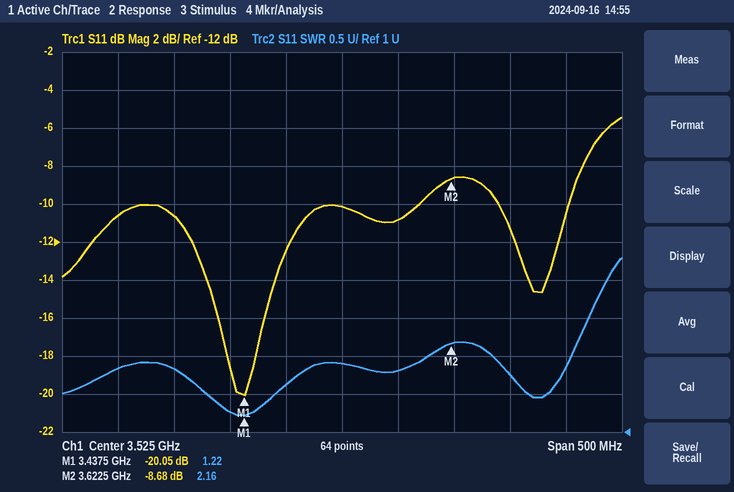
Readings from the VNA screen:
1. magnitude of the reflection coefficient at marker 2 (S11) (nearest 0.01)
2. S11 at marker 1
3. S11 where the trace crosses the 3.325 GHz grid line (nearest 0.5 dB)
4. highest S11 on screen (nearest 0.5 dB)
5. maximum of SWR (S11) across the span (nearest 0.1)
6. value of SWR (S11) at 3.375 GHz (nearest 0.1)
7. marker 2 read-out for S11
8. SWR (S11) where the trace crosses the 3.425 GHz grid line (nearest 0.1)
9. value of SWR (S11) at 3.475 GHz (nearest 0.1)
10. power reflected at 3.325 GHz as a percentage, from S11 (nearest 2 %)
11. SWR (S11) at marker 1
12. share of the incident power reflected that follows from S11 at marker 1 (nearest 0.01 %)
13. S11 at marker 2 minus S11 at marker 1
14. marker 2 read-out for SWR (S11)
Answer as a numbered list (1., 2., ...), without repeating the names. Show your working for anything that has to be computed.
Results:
1. 10^(-8.68/20) ≈ 0.37
2. -20.05 dB
3. -10.5 dB
4. -5.5 dB
5. 3.3
6. 1.8
7. -8.68 dB
8. 1.3
9. 1.6
10. 10^(-10.5/10) ≈ 8.91 %, so 8 % to the nearest 2 %
11. 1.22
12. 10^(-20.05/10) ≈ 0.99 %
13. -8.68 − (-20.05) = 11.37 dB
14. 2.16
